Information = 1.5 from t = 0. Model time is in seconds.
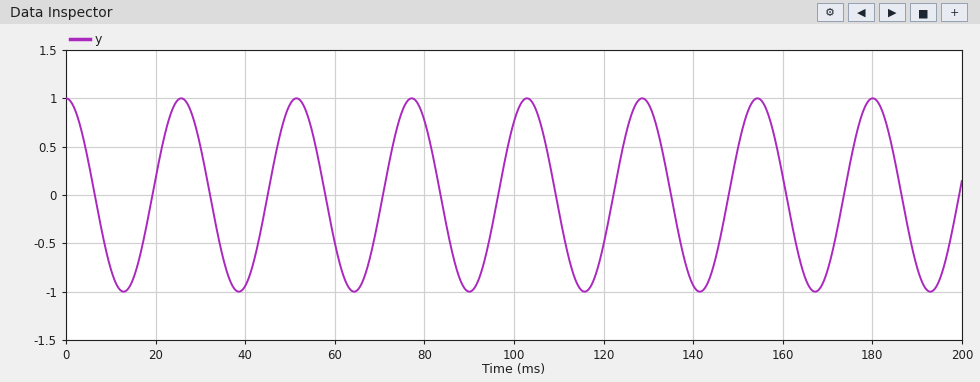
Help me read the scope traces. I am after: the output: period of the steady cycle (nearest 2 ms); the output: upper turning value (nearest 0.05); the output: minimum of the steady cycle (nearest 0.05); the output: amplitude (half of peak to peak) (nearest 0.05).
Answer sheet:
26 ms
1.00
-1.00
1.00
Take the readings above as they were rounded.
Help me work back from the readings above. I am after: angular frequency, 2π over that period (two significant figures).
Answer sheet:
0.24 rad/ms
